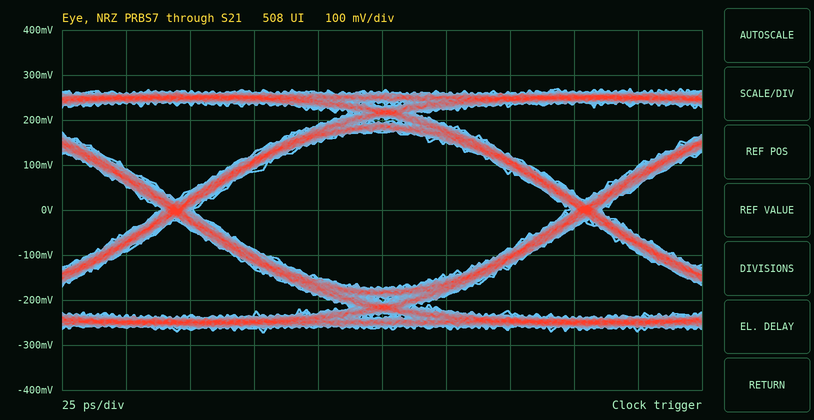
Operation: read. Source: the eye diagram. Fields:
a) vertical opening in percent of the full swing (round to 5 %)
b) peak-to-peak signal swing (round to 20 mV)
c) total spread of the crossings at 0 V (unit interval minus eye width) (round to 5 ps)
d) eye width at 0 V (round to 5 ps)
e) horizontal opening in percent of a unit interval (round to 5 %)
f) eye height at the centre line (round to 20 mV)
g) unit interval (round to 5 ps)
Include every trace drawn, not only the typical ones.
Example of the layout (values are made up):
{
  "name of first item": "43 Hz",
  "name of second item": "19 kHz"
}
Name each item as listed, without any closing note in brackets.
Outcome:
{
  "vertical opening in percent of the full swing": "65 %",
  "peak-to-peak signal swing": "540 mV",
  "total spread of the crossings at 0 V (unit interval minus eye width)": "15 ps",
  "eye width at 0 V": "145 ps",
  "horizontal opening in percent of a unit interval": "90 %",
  "eye height at the centre line": "340 mV",
  "unit interval": "160 ps"
}
